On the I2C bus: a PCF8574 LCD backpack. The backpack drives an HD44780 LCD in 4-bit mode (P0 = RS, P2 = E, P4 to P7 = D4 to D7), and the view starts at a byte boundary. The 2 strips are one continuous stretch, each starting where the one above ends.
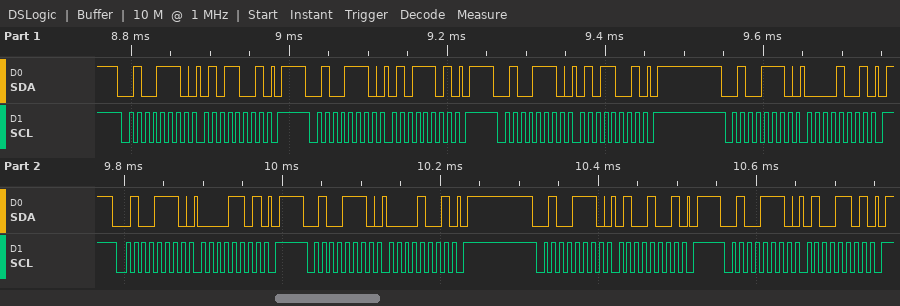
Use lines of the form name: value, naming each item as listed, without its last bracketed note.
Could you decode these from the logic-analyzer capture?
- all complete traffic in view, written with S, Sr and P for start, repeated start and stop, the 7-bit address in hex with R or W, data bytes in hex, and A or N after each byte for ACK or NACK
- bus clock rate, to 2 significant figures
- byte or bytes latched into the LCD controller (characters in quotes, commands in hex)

all complete traffic in view, written with S, Sr and P for start, repeated start and stop, the 7-bit address in hex with R or W, data bytes in hex, and A or N after each byte for ACK or NACK: S 27W A 59 A P S 27W A 5D A P S 27W A 59 A P S 27W A 09 A P S 27W A 0D A P S 27W A 09 A P S 27W A 49 A P S 27W A 4D A P
bus clock rate, to 2 significant figures: 100 kHz
byte or bytes latched into the LCD controller: 'P'
